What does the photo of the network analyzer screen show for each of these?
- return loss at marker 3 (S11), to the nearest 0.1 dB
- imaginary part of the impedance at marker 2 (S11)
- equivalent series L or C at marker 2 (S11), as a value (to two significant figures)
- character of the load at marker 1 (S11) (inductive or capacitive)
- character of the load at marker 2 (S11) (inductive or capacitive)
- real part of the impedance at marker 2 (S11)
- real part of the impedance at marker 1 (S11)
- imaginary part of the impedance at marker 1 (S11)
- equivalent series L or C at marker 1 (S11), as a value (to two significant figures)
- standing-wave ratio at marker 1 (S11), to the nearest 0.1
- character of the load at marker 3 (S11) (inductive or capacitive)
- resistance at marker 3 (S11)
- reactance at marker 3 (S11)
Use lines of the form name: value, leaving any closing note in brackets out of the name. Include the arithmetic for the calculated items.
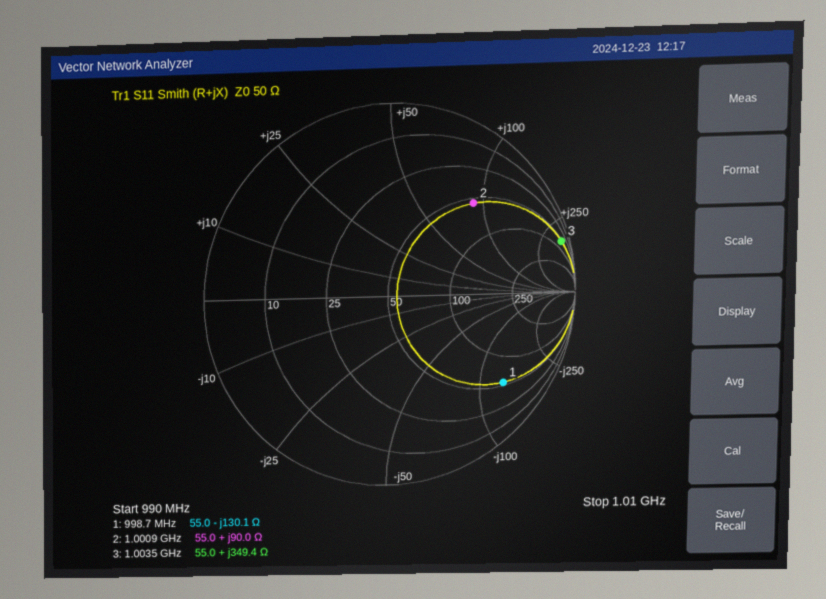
return loss at marker 3 (S11), to the nearest 0.1 dB: 0.4 dB
imaginary part of the impedance at marker 2: +90.0 Ω
equivalent series L or C at marker 2 (S11), as a value: L = 90 Ω/(2π × 1.0009 GHz) ≈ 14 nH
character of the load at marker 1 (S11): capacitive
character of the load at marker 2 (S11): inductive
real part of the impedance at marker 2: 55.0 Ω
real part of the impedance at marker 1: 55.0 Ω
imaginary part of the impedance at marker 1: -130.1 Ω
equivalent series L or C at marker 1 (S11), as a value: C = 1/(2π × 998.7 MHz × 130.1 Ω) ≈ 1.2 pF
standing-wave ratio at marker 1 (S11), to the nearest 0.1: 8.0
character of the load at marker 3 (S11): inductive
resistance at marker 3: 55.0 Ω
reactance at marker 3: +349.4 Ω
